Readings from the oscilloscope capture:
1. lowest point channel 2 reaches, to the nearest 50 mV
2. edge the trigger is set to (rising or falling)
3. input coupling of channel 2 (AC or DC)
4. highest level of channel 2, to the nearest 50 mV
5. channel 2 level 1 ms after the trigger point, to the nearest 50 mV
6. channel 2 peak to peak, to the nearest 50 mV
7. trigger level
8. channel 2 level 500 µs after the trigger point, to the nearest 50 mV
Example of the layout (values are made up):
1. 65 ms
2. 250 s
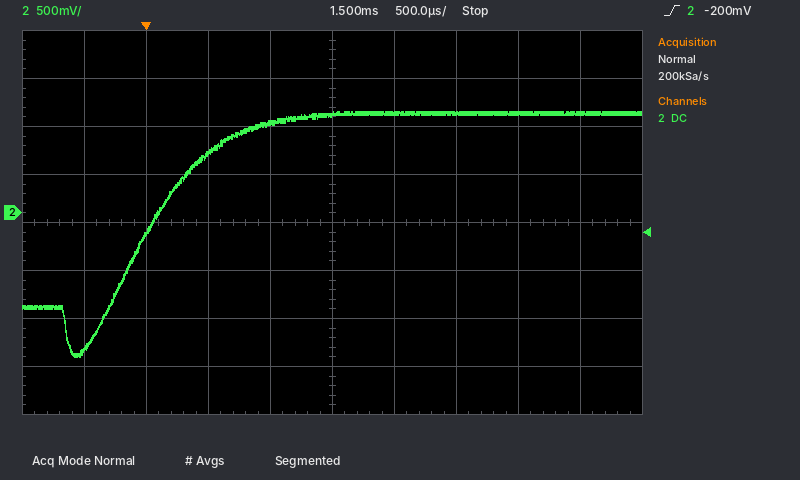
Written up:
1. -1.50 V
2. rising
3. DC
4. 1.05 V
5. 950 mV
6. 2.55 V
7. -200 mV
8. 600 mV
